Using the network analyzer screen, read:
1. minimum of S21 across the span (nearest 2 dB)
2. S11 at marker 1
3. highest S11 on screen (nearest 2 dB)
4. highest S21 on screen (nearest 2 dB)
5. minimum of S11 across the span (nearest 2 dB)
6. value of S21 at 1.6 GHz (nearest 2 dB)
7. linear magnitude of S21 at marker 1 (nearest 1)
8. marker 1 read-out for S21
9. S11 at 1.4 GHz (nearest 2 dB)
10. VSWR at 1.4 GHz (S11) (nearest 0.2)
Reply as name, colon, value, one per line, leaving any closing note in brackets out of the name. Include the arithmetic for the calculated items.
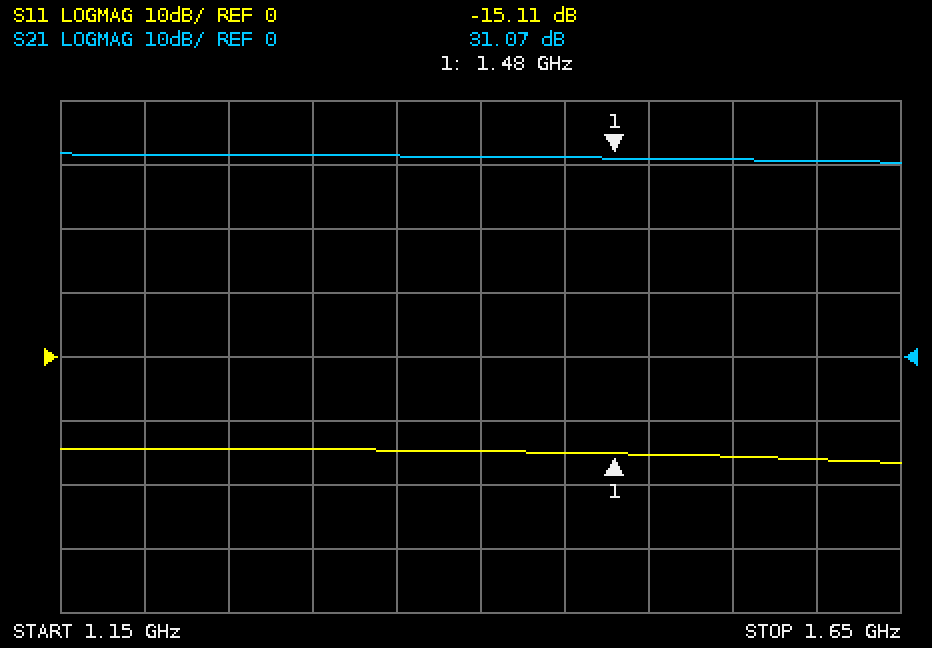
minimum of S21 across the span: 30 dB
S11 at marker 1: -15.11 dB
highest S11 on screen: -14 dB
highest S21 on screen: 32 dB
minimum of S11 across the span: -16 dB
value of S21 at 1.6 GHz: 30 dB
linear magnitude of S21 at marker 1: 10^(31.07/20) ≈ 36
marker 1 read-out for S21: 31.07 dB
S11 at 1.4 GHz: -14 dB
VSWR at 1.4 GHz (S11): |Γ| = 10^(-14/20) = 0.1995; VSWR = (1 + 0.1995)/(1 − 0.1995) ≈ 1.50, so 1.4 to the nearest 0.2
